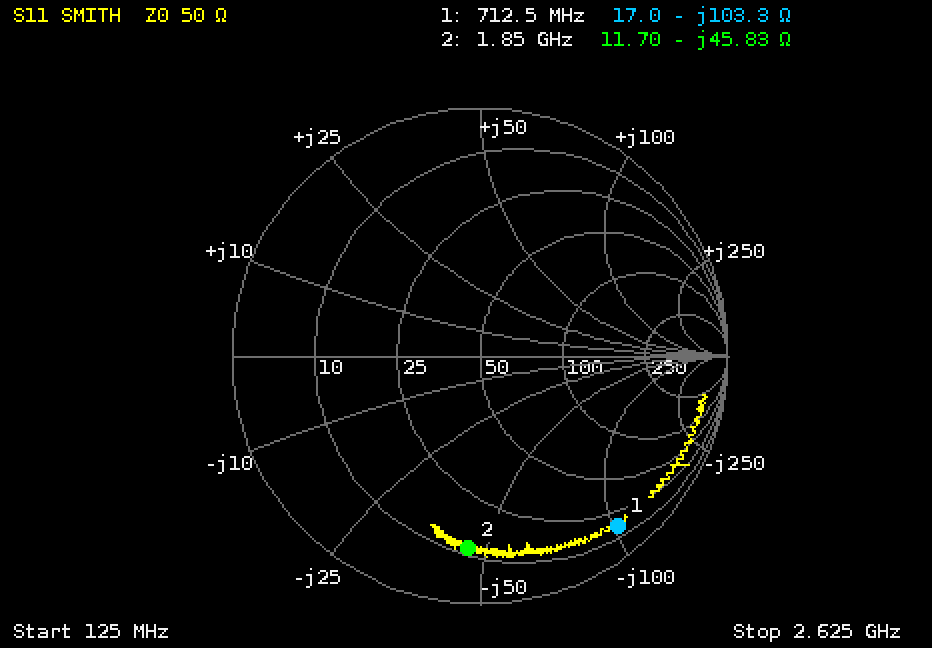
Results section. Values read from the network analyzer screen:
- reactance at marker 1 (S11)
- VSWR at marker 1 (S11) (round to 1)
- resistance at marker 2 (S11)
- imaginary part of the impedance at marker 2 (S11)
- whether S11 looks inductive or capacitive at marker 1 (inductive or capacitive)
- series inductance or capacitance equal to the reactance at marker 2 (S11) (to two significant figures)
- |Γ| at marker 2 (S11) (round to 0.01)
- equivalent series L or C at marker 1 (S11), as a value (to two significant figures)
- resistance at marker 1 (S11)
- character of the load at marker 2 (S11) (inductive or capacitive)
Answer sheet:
-103.3 Ω
16
11.70 Ω
-45.83 Ω
capacitive
1.9 pF
0.78
2.2 pF
17.0 Ω
capacitive
